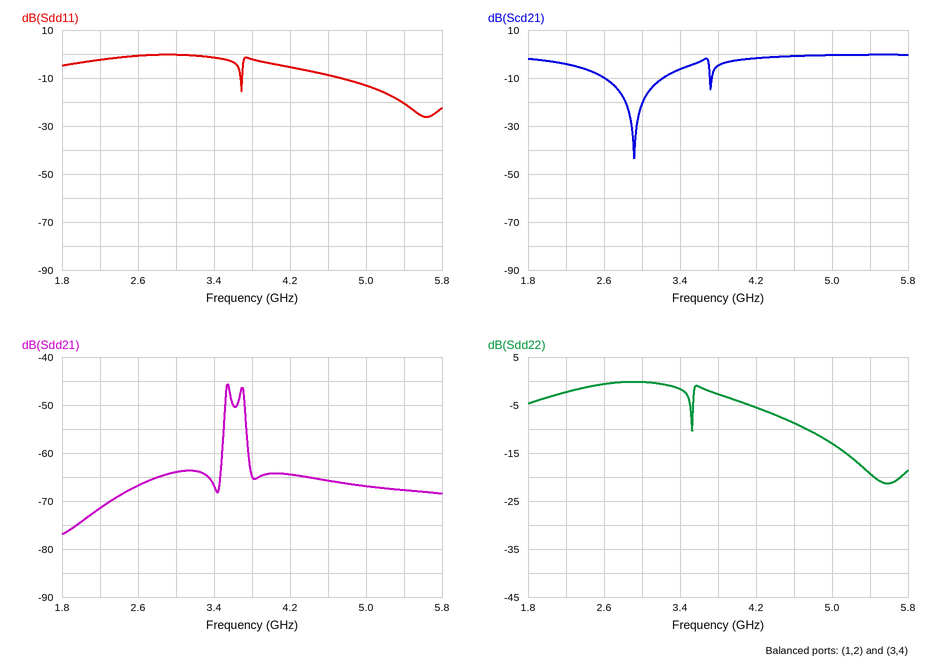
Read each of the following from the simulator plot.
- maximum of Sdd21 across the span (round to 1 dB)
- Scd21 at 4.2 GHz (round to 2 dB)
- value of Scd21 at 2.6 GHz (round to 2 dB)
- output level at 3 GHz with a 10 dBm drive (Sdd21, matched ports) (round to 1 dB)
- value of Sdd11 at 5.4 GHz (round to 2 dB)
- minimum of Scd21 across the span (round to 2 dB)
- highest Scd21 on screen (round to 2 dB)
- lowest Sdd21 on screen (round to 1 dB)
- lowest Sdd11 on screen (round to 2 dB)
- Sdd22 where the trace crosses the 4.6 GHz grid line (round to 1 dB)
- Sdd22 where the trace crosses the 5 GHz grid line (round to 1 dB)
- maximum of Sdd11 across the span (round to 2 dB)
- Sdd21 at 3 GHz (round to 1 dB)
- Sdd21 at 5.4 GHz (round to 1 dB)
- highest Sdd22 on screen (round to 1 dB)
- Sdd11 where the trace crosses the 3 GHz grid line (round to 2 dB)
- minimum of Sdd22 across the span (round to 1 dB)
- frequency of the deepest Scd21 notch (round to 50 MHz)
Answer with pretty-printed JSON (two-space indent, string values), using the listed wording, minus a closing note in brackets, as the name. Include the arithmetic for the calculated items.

{
  "maximum of Sdd21 across the span": "-46 dB",
  "Scd21 at 4.2 GHz": "-2 dB",
  "value of Scd21 at 2.6 GHz": "-10 dB",
  "output level at 3 GHz with a 10 dBm drive (Sdd21, matched ports)": "10 dBm + (-64 dB) = -54 dBm",
  "value of Sdd11 at 5.4 GHz": "-20 dB",
  "minimum of Scd21 across the span": "-44 dB",
  "highest Scd21 on screen": "0 dB",
  "lowest Sdd21 on screen": "-77 dB",
  "lowest Sdd11 on screen": "-26 dB",
  "Sdd22 where the trace crosses the 4.6 GHz grid line": "-9 dB",
  "Sdd22 where the trace crosses the 5 GHz grid line": "-13 dB",
  "maximum of Sdd11 across the span": "0 dB",
  "Sdd21 at 3 GHz": "-64 dB",
  "Sdd21 at 5.4 GHz": "-68 dB",
  "highest Sdd22 on screen": "0 dB",
  "Sdd11 where the trace crosses the 3 GHz grid line": "0 dB",
  "minimum of Sdd22 across the span": "-21 dB",
  "frequency of the deepest Scd21 notch": "2.90 GHz"
}
